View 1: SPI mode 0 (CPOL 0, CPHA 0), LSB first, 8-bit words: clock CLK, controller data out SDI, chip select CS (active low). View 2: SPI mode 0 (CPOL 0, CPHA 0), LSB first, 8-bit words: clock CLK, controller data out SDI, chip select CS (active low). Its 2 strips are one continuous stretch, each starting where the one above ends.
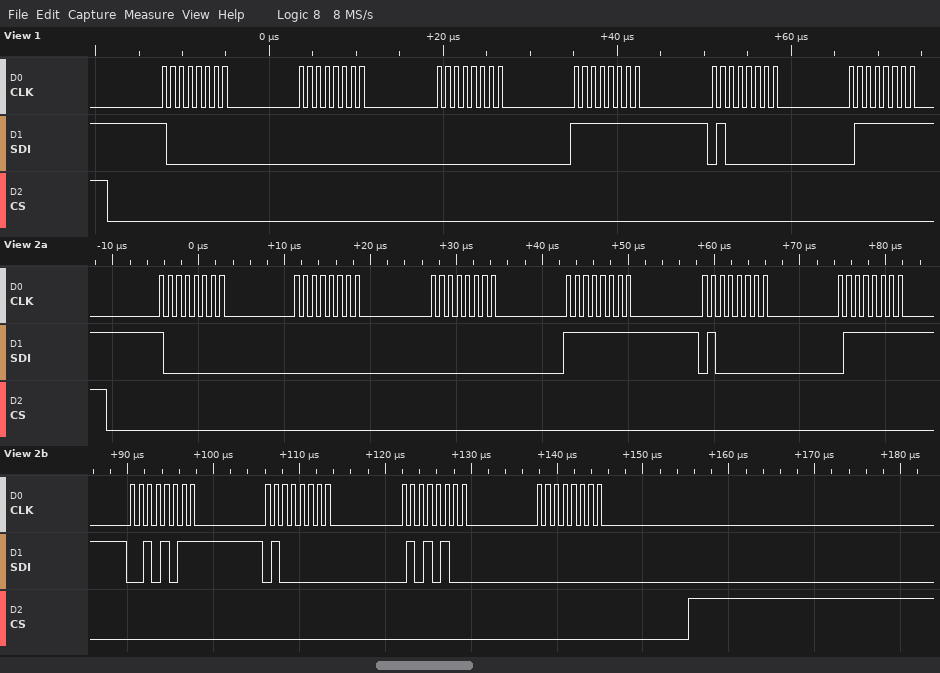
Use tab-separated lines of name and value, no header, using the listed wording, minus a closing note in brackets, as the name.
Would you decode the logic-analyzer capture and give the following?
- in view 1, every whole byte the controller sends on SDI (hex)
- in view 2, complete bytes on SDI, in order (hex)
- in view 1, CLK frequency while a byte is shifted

in view 1, every whole byte the controller sends on SDI	01 00 00 FF 02 FE
in view 2, complete bytes on SDI, in order	01 00 00 FF 02 FE D4 02 2A 00
in view 1, CLK frequency while a byte is shifted	1 MHz
